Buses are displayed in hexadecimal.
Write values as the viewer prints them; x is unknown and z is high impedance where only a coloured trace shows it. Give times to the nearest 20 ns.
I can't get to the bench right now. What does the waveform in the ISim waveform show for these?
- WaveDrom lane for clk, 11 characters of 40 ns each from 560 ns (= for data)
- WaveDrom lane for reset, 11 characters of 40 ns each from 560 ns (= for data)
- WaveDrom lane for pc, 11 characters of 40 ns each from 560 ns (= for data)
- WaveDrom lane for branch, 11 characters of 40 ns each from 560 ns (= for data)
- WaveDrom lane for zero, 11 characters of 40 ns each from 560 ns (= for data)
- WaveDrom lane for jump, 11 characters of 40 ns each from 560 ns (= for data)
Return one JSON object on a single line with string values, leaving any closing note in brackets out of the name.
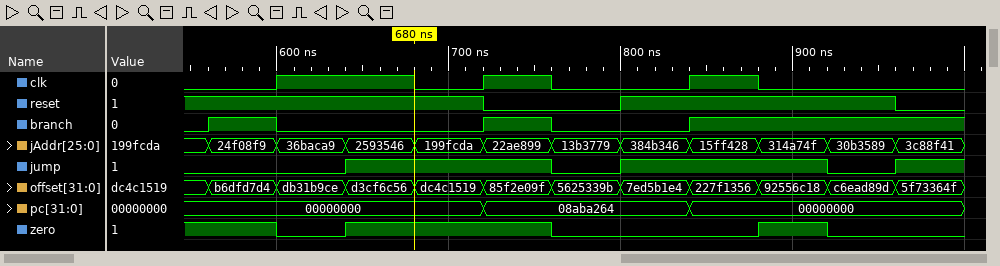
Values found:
{"WaveDrom lane for clk, 11 characters of 40 ns each from 560 ns": "{name: 'clk', wave: '01.010.10..'}", "WaveDrom lane for reset, 11 characters of 40 ns each from 560 ns": "{name: 'reset', wave: '1...0.1...0'}", "WaveDrom lane for pc, 11 characters of 40 ns each from 560 ns": "{name: 'pc', wave: '=...=..=...', data: '00000000 08aba264 00000000'}", "WaveDrom lane for branch, 11 characters of 40 ns each from 560 ns": "{name: 'branch', wave: '10..10.1...'}", "WaveDrom lane for zero, 11 characters of 40 ns each from 560 ns": "{name: 'zero', wave: '101..0..10.'}", "WaveDrom lane for jump, 11 characters of 40 ns each from 560 ns": "{name: 'jump', wave: '0.1..01..01'}"}
